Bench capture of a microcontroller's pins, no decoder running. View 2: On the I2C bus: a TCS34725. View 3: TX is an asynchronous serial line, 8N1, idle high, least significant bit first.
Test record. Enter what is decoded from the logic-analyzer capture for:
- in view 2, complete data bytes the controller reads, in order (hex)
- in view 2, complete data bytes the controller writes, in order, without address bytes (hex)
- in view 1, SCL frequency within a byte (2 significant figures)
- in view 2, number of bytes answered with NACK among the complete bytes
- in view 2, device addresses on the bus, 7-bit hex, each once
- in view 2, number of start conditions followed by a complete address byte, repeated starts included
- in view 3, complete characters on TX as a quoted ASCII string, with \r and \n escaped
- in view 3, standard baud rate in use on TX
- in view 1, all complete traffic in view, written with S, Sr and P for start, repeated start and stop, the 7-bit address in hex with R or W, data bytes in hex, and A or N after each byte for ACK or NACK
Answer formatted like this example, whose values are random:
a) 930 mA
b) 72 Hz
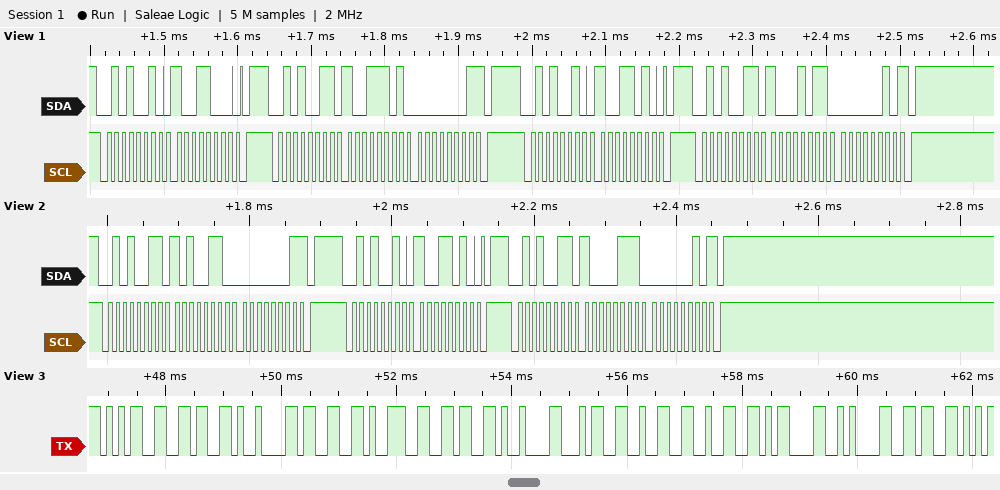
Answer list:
a) A6 01 87 02
b) 9A
c) 100 kHz
d) 2
e) 0x29
f) 3
g) "56\t396\t422\r\n6"
h) 9600 baud
i) S 29W A 98 A P S 29R A 9D A 01 N P S 29W A 9A A P S 29R A 8B A 02 N P
